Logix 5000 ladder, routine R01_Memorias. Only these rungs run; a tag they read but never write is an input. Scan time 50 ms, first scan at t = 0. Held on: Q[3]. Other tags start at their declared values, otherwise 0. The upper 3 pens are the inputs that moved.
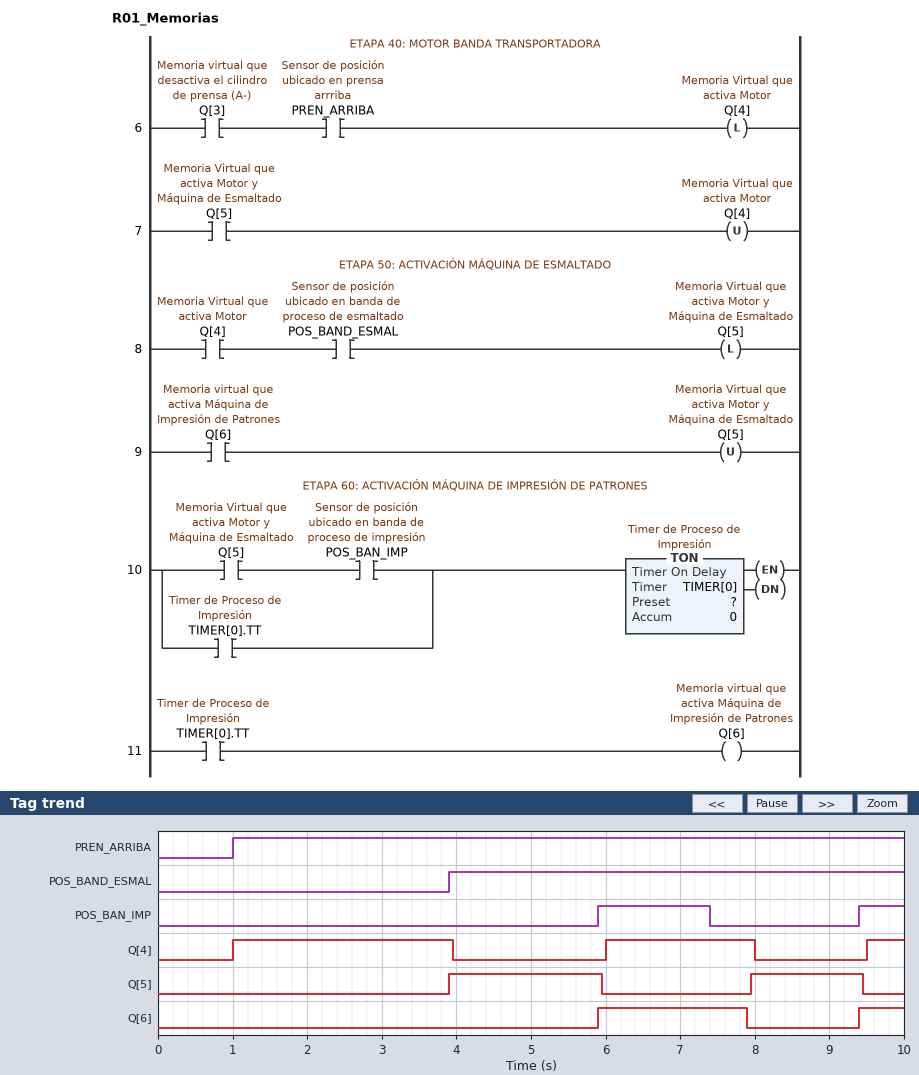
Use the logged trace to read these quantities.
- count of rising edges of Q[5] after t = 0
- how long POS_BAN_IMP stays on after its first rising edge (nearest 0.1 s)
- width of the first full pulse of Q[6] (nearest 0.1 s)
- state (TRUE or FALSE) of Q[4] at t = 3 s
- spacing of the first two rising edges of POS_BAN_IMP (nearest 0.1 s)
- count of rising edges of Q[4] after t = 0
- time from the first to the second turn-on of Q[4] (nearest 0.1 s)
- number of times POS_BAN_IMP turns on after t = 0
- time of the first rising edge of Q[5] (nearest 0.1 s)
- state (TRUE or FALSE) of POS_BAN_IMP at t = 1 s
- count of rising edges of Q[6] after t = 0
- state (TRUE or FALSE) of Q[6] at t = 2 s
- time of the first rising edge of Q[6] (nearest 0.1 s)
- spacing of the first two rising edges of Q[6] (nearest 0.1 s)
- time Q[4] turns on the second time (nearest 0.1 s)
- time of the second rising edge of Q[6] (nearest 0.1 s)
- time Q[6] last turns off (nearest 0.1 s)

2
1.5 s
2.0 s
TRUE
3.5 s
3
5.0 s
2
3.9 s
FALSE
2
FALSE
5.9 s
3.5 s
6.0 s
9.4 s
7.9 s
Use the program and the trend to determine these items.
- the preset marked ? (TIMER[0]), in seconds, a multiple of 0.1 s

2.0 s
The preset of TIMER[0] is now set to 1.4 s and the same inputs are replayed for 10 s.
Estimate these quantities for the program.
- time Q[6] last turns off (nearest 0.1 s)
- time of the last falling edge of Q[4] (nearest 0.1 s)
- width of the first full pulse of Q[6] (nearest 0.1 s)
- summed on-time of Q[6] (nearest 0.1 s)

7.3 s
7.4 s
1.4 s
2.0 s
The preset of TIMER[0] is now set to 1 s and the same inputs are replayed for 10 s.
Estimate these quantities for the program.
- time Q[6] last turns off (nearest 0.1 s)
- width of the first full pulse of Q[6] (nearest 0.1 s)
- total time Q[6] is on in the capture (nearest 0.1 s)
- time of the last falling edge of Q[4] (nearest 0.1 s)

6.9 s
1.0 s
1.6 s
7.0 s
